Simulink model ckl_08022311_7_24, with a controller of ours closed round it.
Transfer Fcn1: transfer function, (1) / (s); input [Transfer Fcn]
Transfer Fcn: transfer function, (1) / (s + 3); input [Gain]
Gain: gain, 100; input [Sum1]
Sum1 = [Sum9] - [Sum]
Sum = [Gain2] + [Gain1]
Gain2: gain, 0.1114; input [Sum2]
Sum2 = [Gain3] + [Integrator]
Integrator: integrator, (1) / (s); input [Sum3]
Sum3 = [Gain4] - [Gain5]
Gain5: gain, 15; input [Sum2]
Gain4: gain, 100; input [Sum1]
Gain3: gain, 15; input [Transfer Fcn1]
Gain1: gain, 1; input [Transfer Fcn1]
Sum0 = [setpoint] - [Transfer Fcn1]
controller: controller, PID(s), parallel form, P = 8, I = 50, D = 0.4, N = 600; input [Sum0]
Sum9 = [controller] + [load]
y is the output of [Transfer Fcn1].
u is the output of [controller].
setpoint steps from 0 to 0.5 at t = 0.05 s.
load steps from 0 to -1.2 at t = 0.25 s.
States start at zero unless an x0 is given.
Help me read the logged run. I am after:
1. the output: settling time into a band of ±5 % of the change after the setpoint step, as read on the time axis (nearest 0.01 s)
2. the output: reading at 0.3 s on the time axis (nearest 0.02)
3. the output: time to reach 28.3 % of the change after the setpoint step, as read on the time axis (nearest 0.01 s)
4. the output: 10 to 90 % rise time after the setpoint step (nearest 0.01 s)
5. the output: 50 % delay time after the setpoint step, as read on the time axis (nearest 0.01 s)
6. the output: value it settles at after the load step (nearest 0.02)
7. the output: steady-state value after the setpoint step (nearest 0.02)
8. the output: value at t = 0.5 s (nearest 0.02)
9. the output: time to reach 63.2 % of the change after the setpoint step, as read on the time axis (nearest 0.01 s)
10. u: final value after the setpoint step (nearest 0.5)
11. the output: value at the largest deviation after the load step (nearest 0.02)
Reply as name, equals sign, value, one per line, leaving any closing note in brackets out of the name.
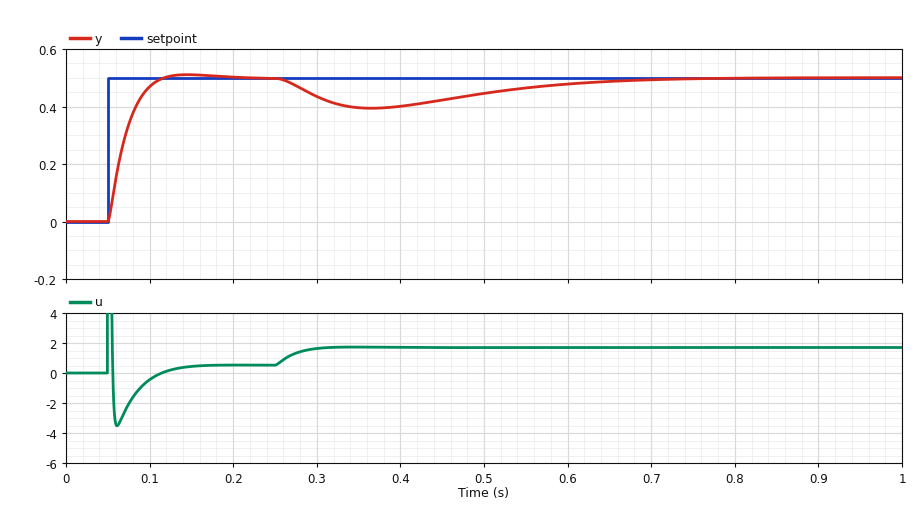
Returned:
the output: settling time into a band of ±5 % of the change after the setpoint step, as read on the time axis = 0.10 s
the output: reading at 0.3 s on the time axis = 0.44
the output: time to reach 28.3 % of the change after the setpoint step, as read on the time axis = 0.06 s
the output: 10 to 90 % rise time after the setpoint step = 0.04 s
the output: 50 % delay time after the setpoint step, as read on the time axis = 0.07 s
the output: value it settles at after the load step = 0.50
the output: steady-state value after the setpoint step = 0.50
the output: value at t = 0.5 s = 0.44
the output: time to reach 63.2 % of the change after the setpoint step, as read on the time axis = 0.07 s
u: final value after the setpoint step = 0.5
the output: value at the largest deviation after the load step = 0.40
